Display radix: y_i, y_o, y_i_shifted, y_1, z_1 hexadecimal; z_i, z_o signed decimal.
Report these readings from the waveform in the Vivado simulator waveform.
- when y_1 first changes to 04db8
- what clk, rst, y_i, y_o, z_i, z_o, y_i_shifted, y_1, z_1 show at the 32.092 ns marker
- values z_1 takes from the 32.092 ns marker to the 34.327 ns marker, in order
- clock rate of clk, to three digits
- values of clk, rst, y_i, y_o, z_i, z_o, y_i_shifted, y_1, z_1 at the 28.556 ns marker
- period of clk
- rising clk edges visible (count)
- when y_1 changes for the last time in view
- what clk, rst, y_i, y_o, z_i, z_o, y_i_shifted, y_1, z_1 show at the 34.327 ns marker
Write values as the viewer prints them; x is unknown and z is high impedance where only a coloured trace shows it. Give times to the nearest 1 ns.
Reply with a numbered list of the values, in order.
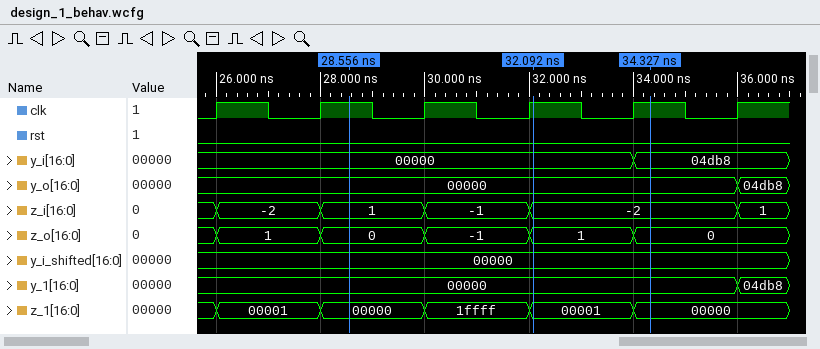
1. 36 ns
2. clk=1, rst=0, y_i=00000, y_o=00000, z_i=-2, z_o=1, y_i_shifted=00000, y_1=00000, z_1=00001
3. 00001, 00000
4. 500 MHz
5. clk=1, rst=0, y_i=00000, y_o=00000, z_i=1, z_o=0, y_i_shifted=00000, y_1=00000, z_1=00000
6. 2 ns
7. 6
8. 36 ns
9. clk=1, rst=0, y_i=04db8, y_o=00000, z_i=-2, z_o=0, y_i_shifted=00000, y_1=00000, z_1=00000
